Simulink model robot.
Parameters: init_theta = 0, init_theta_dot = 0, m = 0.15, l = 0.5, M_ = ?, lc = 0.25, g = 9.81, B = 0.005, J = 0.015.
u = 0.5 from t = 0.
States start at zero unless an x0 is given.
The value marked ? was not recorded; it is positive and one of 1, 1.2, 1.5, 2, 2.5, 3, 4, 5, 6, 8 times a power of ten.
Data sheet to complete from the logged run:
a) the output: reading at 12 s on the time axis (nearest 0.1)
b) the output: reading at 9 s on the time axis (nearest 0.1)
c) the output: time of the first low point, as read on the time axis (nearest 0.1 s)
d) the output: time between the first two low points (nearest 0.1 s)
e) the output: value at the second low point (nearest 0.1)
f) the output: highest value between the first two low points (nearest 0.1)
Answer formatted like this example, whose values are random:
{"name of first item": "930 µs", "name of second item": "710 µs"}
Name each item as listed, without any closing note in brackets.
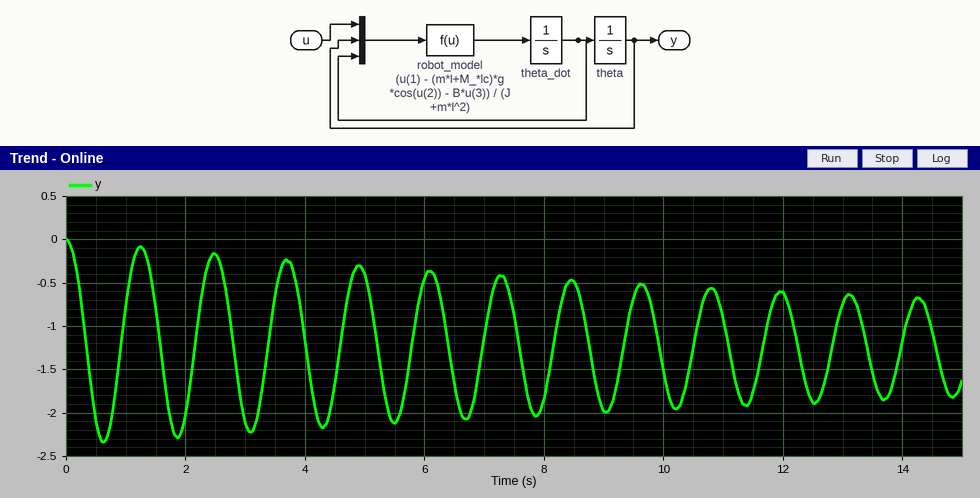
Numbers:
{"the output: reading at 12 s on the time axis": "-0.6", "the output: reading at 9 s on the time axis": "-2.0", "the output: time of the first low point, as read on the time axis": "0.6 s", "the output: time between the first two low points": "1.2 s", "the output: value at the second low point": "-2.3", "the output: highest value between the first two low points": "-0.1"}
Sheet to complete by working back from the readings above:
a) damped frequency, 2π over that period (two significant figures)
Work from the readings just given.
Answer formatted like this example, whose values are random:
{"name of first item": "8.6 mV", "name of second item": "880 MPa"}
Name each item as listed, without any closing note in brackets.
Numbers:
{"damped frequency, 2π over that period": "5.2 rad/s"}
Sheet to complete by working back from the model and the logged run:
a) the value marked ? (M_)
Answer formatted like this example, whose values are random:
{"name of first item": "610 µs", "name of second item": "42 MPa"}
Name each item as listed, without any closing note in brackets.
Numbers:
{"the value marked ?": "0.4"}
